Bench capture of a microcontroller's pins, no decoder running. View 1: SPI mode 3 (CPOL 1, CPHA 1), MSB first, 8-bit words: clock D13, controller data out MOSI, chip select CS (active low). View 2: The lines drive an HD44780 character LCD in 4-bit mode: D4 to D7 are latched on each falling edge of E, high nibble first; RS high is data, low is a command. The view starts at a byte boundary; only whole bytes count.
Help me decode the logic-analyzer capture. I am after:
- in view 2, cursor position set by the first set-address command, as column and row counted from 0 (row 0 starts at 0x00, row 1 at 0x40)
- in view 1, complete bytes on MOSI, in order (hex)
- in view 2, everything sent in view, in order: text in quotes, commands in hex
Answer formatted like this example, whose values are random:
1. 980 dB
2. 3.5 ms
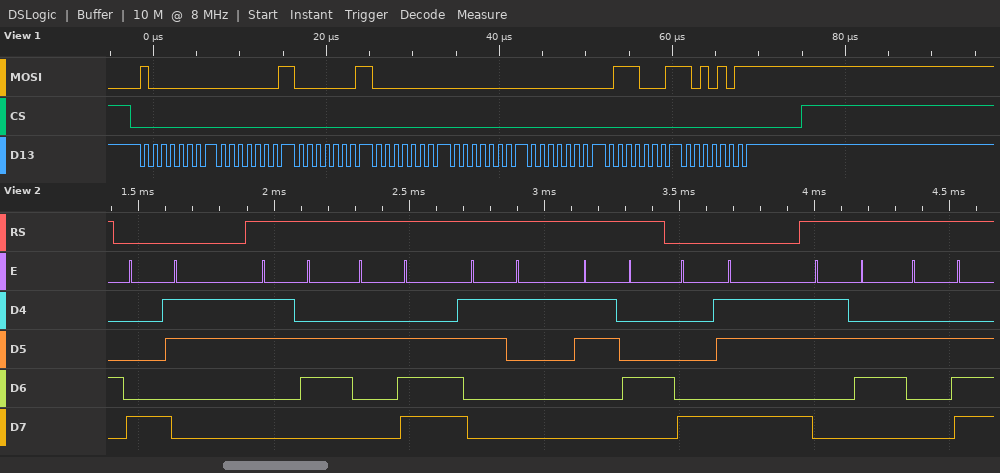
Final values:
1. column 3, row 0
2. 80 01 01 00 00 00 71 AB
3. 0x83 "6.14" 0x8B "6."
